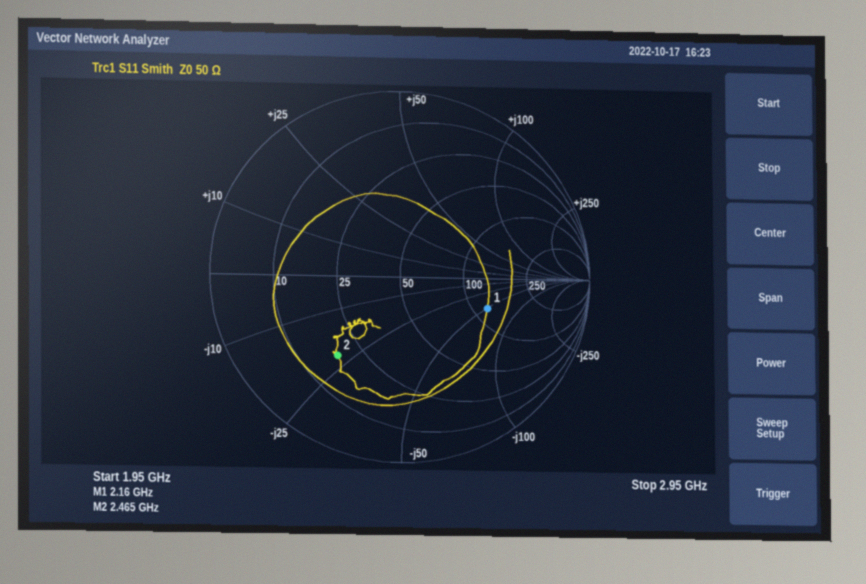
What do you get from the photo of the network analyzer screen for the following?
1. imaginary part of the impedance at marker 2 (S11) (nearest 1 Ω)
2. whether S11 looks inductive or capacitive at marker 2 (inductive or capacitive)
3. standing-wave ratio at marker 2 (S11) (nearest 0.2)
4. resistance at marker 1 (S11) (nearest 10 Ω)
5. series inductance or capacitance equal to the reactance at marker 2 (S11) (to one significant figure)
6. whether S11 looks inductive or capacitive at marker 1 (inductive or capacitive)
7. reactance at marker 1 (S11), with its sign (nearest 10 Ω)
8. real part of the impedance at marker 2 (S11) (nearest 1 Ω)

-22 Ω
capacitive
3.4
120 Ω
3 pF
capacitive
-50 Ω
18 Ω
